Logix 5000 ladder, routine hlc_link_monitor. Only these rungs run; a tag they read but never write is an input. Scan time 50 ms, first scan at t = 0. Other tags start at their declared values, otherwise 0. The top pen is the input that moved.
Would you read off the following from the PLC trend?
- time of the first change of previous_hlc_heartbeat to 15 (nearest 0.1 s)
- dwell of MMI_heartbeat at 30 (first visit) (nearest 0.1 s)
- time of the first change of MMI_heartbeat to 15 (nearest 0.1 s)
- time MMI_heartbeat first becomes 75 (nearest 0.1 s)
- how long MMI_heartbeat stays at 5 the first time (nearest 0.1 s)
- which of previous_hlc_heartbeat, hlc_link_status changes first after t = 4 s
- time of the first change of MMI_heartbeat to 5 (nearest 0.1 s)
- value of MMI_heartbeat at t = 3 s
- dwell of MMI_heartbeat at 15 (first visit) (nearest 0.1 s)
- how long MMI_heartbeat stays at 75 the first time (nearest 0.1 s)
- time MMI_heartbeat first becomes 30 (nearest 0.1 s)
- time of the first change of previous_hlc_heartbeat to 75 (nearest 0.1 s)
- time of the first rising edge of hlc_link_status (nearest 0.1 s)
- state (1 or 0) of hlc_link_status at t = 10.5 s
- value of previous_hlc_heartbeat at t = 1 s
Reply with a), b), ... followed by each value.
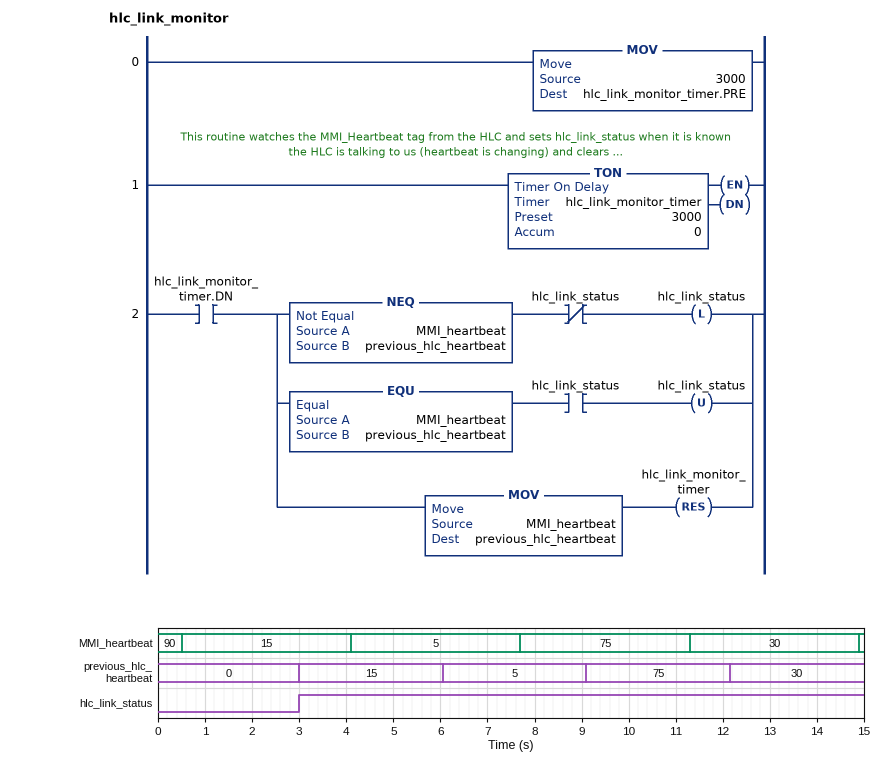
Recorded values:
a) 3.0 s
b) 3.6 s
c) 0.5 s
d) 7.7 s
e) 3.6 s
f) previous_hlc_heartbeat
g) 4.1 s
h) 15
i) 3.6 s
j) 3.6 s
k) 11.3 s
l) 9.1 s
m) 3.0 s
n) 1
o) 0
